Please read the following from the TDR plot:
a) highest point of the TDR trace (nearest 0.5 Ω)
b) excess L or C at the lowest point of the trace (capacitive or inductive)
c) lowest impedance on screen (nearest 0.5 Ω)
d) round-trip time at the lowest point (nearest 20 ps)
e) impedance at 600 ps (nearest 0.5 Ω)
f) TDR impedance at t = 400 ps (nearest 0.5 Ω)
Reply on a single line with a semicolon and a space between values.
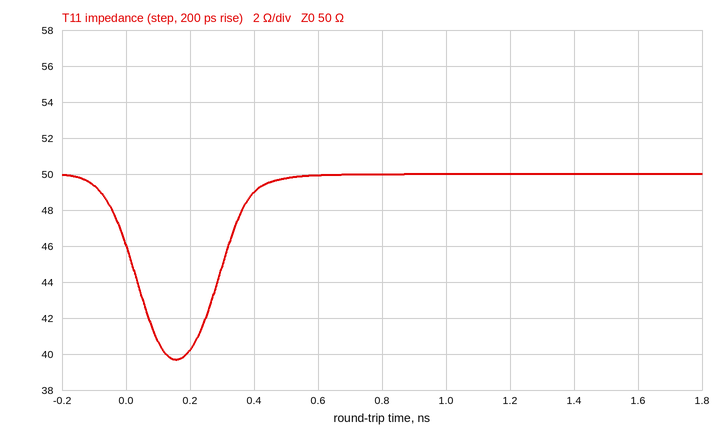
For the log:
50.0 Ω; capacitive; 39.5 Ω; 160 ps; 50.0 Ω; 49.0 Ω
